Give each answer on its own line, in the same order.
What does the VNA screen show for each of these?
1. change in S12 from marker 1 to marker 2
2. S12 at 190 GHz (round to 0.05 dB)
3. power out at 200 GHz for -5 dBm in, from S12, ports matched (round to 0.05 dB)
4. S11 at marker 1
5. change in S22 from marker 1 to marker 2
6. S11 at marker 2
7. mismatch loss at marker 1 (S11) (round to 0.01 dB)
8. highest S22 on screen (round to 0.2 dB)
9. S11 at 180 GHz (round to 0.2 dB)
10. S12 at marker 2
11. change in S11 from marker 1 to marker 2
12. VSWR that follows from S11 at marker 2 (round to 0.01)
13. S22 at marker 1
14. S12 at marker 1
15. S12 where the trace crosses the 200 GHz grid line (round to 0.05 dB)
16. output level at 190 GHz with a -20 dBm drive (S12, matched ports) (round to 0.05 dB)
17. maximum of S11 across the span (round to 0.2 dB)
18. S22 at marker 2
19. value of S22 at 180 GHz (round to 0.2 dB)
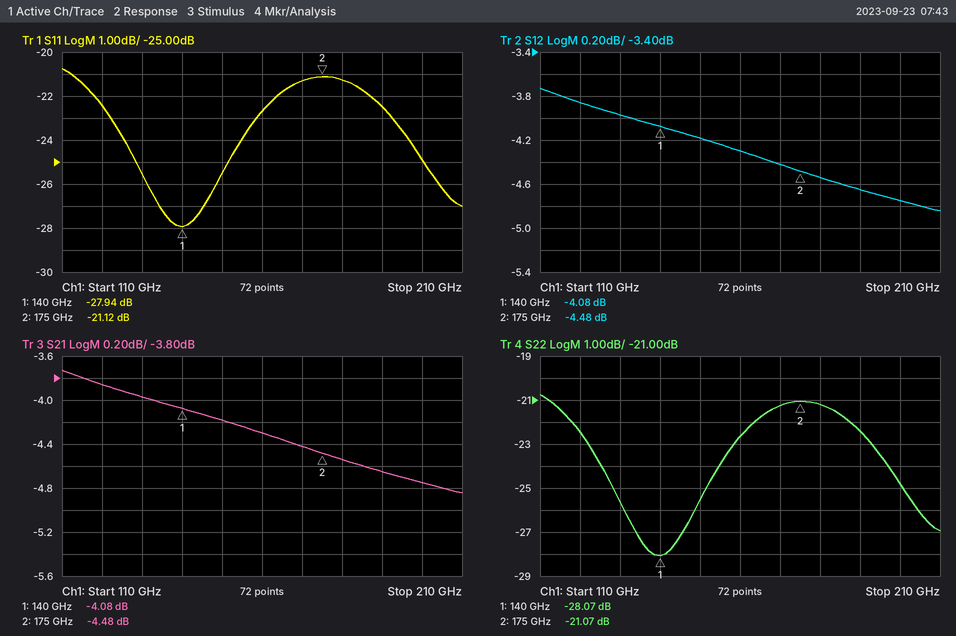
-0.40 dB
-4.65 dB
-9.75 dBm
-27.94 dB
7.00 dB
-21.12 dB
0.01 dB
-20.8 dB
-21.2 dB
-4.48 dB
6.82 dB
1.19
-28.07 dB
-4.08 dB
-4.75 dB
-24.65 dBm
-20.8 dB
-21.07 dB
-21.2 dB
